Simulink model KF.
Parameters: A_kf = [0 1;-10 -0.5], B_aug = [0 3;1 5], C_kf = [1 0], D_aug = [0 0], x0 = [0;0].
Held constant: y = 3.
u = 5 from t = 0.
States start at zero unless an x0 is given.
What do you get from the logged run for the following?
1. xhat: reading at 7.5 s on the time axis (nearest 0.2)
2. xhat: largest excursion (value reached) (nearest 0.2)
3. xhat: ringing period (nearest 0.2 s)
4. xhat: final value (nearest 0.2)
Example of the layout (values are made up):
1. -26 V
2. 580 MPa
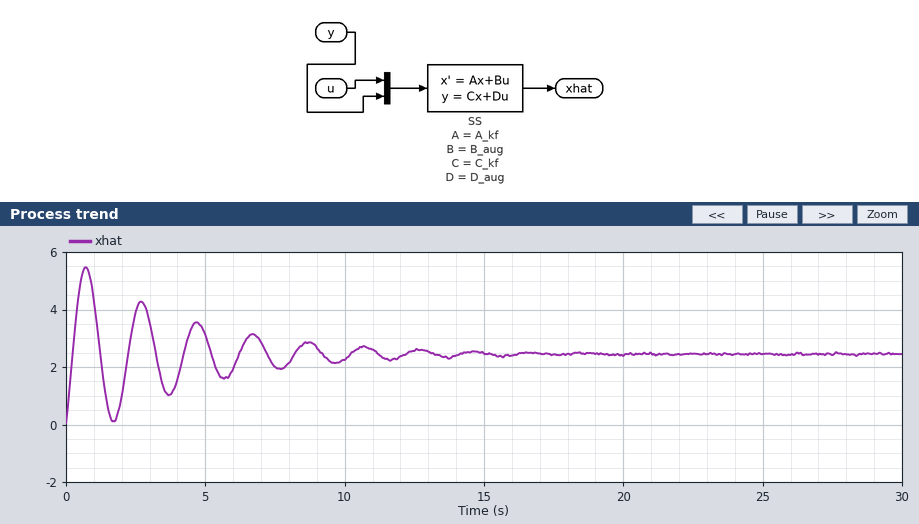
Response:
1. 2.0
2. 5.4
3. 2.0 s
4. 2.4
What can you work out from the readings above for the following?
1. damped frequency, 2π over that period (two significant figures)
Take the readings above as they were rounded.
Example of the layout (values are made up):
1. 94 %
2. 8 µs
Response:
1. 3.1 rad/s
